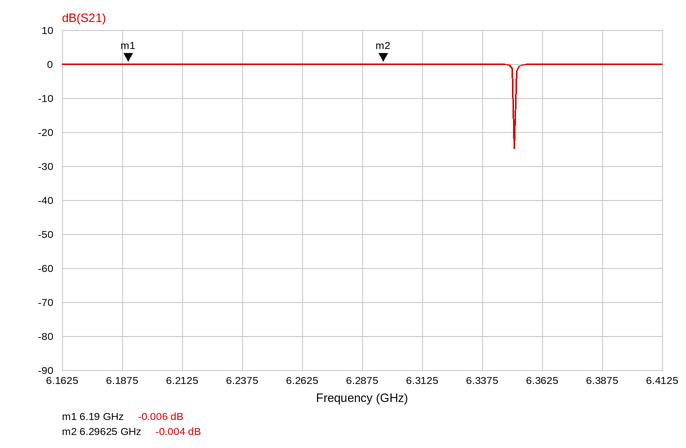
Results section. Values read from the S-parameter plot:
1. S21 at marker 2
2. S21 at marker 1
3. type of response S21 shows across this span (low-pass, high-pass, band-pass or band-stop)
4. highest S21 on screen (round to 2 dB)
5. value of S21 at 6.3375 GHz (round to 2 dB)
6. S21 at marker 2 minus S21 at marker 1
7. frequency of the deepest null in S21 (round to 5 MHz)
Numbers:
-0.004 dB
-0.006 dB
band-stop
0 dB
0 dB
0.002 dB
6.350 GHz
